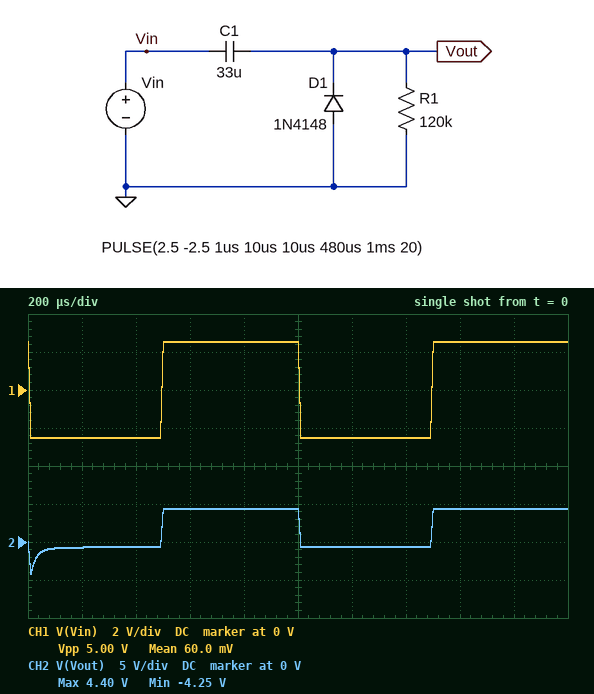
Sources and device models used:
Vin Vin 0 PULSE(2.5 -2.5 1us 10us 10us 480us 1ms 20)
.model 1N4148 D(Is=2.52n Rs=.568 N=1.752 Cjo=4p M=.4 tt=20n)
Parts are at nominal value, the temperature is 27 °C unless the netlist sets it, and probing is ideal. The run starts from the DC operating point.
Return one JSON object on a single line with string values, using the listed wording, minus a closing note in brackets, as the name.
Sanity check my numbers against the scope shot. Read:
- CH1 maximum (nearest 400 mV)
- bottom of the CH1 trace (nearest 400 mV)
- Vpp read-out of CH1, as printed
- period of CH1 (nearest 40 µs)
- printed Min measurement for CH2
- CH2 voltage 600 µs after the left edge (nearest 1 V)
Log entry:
{"CH1 maximum": "2.4 V", "bottom of the CH1 trace": "-2.4 V", "Vpp read-out of CH1, as printed": "5.00 V", "period of CH1": "1.00 ms", "printed Min measurement for CH2": "-4.25 V", "CH2 voltage 600 µs after the left edge": "4 V"}
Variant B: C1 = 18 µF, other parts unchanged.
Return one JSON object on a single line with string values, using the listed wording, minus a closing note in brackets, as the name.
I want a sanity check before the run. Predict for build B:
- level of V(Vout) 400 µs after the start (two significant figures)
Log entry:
{"level of V(Vout) 400 µs after the start": "-630 mV"}
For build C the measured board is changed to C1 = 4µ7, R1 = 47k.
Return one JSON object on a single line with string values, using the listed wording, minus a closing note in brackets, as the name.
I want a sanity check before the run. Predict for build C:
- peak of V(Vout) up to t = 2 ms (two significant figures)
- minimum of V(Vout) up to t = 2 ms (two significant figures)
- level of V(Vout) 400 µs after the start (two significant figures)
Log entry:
{"peak of V(Vout) up to t = 2 ms": "4.5 V", "minimum of V(Vout) up to t = 2 ms": "-2.2 V", "level of V(Vout) 400 µs after the start": "-560 mV"}
